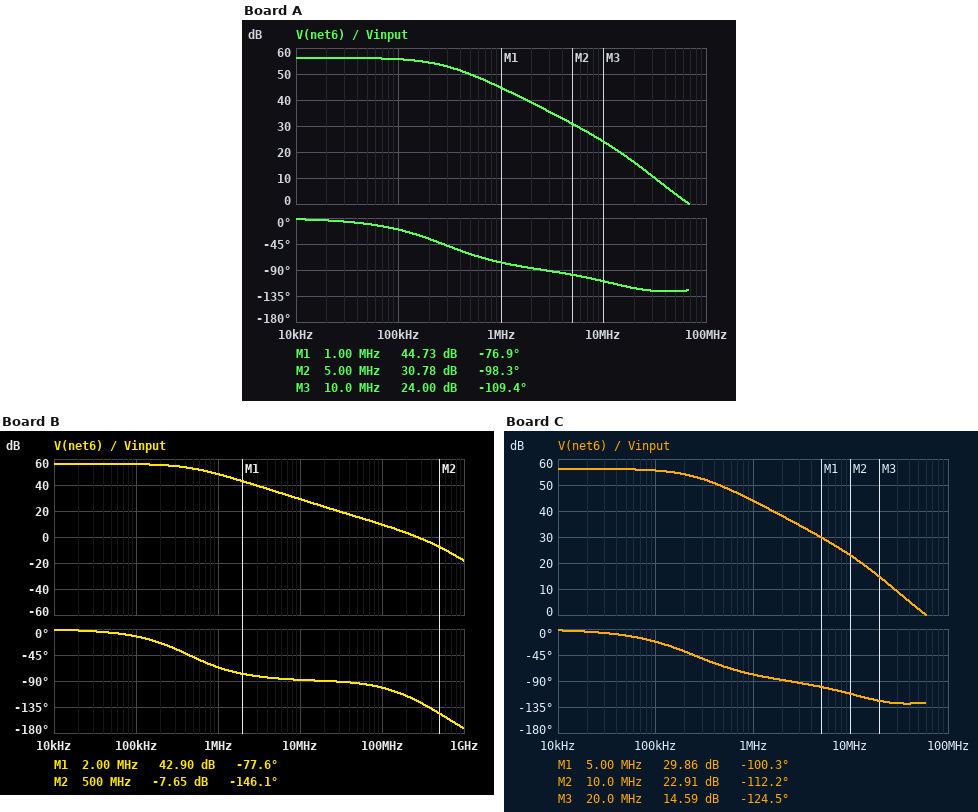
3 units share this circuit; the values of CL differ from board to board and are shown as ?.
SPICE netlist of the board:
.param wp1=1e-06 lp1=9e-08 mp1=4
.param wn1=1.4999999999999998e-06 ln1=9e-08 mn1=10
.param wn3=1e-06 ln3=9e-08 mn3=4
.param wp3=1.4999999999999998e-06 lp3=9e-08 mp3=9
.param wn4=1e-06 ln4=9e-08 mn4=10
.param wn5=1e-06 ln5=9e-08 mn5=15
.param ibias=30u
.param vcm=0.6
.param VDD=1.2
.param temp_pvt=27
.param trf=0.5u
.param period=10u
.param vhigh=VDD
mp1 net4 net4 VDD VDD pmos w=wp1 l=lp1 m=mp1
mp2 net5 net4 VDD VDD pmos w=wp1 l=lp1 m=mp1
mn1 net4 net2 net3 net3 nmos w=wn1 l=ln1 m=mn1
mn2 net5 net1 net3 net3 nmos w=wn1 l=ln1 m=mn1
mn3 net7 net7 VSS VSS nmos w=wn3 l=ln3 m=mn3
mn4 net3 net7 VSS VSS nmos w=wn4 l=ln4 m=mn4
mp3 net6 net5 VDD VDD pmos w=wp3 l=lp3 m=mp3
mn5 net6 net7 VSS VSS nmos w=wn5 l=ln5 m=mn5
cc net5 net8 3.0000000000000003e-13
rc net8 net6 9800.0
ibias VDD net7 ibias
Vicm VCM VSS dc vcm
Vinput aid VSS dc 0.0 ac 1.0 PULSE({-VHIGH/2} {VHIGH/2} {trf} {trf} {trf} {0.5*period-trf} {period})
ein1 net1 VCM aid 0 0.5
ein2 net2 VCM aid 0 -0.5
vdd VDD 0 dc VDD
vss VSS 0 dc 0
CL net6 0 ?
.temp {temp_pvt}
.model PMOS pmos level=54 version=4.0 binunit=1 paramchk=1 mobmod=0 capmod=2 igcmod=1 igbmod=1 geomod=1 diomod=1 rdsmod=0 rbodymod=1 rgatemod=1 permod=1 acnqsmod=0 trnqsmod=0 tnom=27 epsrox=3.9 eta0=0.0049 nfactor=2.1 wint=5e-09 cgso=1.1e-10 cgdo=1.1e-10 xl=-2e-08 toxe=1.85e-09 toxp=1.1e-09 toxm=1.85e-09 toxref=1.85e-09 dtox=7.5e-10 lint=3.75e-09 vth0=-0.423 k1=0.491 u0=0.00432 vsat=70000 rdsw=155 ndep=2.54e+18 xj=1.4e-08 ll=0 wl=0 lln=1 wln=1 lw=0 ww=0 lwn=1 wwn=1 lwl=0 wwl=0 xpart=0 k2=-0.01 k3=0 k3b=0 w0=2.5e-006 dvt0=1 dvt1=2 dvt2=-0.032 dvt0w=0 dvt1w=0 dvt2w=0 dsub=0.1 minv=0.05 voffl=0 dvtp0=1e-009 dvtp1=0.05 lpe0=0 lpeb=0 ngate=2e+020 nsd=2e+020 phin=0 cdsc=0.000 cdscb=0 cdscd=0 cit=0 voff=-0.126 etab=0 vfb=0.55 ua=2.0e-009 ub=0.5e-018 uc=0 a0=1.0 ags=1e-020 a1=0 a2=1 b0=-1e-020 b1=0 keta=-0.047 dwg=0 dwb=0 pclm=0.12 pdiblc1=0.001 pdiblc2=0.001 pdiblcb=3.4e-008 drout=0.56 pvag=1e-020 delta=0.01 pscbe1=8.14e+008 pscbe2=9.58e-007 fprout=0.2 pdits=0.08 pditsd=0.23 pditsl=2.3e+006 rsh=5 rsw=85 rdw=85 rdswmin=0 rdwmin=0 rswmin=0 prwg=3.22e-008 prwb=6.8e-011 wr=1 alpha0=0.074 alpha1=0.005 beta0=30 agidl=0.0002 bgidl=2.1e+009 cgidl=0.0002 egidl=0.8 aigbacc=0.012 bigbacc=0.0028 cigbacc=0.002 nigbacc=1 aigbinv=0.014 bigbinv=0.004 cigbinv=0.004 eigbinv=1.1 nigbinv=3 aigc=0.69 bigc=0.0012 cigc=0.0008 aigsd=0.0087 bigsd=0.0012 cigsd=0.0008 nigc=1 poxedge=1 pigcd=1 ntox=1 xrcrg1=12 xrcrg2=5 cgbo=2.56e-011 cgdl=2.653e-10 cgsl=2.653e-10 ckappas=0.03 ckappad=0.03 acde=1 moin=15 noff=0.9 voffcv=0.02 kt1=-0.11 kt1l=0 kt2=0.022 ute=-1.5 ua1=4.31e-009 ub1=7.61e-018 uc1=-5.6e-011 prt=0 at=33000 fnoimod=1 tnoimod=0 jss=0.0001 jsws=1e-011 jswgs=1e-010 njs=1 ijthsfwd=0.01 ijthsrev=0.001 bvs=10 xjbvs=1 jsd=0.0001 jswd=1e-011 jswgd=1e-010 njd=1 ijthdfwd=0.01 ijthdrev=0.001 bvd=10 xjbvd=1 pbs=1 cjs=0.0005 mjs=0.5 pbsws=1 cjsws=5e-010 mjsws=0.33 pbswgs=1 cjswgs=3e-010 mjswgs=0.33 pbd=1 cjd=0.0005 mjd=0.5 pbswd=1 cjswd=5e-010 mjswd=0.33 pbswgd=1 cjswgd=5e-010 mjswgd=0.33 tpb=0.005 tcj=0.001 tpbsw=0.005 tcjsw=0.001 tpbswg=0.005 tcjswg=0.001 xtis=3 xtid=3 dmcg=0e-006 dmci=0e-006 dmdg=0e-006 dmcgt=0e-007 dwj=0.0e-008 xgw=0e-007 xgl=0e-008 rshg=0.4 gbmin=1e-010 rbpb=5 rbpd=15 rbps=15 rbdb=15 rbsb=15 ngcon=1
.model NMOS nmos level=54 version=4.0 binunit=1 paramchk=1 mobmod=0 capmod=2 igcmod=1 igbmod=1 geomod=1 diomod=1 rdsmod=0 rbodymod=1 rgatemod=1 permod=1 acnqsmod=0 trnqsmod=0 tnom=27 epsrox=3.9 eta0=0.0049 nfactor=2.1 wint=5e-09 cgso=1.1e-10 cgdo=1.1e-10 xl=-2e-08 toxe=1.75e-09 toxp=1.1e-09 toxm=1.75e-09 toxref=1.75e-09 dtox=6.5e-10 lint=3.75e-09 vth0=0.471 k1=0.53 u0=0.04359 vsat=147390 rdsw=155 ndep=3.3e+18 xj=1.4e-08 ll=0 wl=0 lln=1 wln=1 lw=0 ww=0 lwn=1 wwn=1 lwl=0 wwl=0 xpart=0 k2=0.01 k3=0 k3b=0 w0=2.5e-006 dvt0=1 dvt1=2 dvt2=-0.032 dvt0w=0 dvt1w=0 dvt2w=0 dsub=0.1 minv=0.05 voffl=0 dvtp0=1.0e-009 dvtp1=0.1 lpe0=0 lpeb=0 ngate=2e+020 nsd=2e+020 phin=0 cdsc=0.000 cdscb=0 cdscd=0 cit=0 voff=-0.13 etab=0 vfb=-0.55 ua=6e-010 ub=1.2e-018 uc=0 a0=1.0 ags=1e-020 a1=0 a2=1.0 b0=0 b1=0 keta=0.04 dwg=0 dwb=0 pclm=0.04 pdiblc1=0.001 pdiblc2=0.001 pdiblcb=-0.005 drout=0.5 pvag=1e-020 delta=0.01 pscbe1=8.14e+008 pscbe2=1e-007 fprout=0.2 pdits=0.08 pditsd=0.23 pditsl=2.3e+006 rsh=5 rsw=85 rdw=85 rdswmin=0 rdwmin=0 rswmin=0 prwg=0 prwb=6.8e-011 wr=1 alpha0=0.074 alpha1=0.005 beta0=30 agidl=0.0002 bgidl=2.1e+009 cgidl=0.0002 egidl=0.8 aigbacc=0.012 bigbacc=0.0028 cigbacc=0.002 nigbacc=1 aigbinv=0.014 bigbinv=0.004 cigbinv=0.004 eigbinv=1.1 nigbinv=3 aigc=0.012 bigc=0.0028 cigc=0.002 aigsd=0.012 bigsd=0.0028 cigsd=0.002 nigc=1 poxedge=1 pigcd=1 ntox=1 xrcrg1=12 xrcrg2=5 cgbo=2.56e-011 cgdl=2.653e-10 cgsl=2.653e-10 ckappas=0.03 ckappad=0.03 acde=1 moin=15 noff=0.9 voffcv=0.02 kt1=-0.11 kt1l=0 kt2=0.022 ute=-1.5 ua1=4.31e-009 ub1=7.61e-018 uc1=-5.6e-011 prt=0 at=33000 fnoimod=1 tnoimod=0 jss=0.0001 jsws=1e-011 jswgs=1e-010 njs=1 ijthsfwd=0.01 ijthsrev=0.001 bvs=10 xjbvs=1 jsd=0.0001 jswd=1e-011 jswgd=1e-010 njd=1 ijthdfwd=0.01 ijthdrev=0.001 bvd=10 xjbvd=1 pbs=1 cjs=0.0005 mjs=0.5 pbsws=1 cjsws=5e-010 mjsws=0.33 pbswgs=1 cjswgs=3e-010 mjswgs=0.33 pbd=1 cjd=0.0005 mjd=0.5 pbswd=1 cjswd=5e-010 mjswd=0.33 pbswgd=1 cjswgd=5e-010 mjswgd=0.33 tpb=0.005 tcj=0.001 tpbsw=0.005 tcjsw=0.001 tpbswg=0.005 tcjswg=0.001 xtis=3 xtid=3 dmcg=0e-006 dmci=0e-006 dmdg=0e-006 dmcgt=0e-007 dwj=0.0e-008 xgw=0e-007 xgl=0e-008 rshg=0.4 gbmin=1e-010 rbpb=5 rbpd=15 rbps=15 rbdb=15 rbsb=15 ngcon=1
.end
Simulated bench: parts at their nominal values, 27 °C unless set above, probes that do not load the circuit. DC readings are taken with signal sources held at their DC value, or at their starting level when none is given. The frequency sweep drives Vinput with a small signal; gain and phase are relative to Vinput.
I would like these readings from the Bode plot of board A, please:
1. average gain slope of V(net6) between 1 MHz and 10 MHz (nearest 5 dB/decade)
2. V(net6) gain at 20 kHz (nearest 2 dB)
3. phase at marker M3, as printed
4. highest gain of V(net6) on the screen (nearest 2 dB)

-20 dB/decade
56 dB
-109.4 deg
56 dB
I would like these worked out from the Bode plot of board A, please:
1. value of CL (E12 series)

18 pF
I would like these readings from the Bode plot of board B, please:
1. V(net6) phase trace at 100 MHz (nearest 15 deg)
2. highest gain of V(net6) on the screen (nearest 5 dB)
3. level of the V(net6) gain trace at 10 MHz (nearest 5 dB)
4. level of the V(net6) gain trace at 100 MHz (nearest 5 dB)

-105 deg
55 dB
30 dB
10 dB
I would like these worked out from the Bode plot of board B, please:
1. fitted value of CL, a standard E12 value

3.3 pF
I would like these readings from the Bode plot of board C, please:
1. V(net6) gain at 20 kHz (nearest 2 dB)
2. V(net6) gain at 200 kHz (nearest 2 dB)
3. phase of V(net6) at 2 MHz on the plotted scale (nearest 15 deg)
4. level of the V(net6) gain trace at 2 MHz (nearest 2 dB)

56 dB
54 dB
-90 deg
38 dB
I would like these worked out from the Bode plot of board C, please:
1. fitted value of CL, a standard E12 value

22 pF
